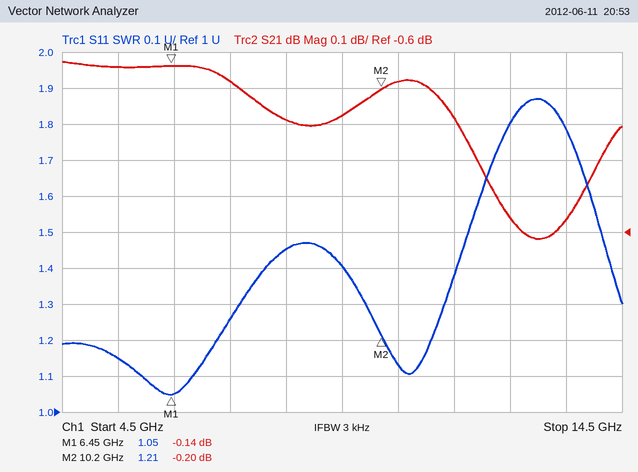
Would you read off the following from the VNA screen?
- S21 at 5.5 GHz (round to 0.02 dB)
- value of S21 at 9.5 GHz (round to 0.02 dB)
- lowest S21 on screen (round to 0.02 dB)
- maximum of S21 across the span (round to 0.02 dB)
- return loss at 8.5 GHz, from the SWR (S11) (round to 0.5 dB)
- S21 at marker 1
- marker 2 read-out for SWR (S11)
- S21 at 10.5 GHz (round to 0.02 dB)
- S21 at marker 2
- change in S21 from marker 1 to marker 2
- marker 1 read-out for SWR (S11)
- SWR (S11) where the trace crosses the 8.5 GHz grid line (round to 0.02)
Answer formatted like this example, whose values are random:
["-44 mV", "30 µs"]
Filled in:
["-0.14 dB", "-0.28 dB", "-0.62 dB", "-0.12 dB", "14.5 dB", "-0.14 dB", "1.21", "-0.18 dB", "-0.20 dB", "-0.06 dB", "1.05", "1.46"]
